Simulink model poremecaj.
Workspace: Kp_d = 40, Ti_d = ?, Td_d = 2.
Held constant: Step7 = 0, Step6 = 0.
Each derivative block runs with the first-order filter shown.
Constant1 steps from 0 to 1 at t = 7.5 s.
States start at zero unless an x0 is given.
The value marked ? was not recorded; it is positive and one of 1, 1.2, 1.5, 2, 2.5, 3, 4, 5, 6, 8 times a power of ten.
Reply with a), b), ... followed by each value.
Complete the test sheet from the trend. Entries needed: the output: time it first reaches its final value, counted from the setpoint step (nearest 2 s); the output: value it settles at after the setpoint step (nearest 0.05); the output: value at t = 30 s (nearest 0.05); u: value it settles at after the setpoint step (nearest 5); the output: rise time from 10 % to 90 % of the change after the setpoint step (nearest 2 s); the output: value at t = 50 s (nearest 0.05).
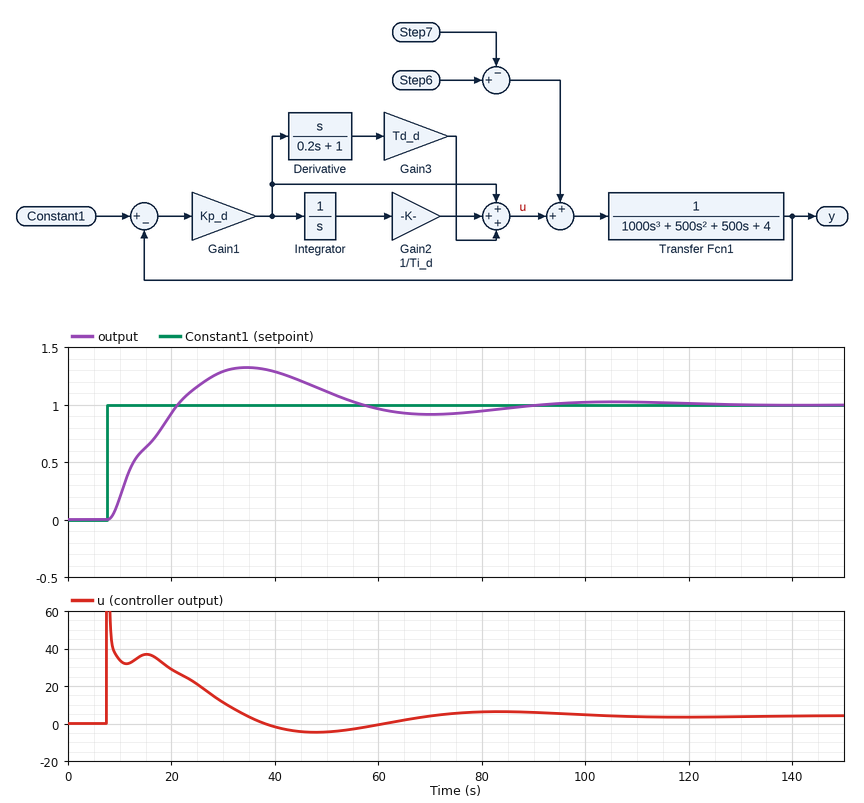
a) 14 s
b) 1.00
c) 1.30
d) 5
e) 10 s
f) 1.10
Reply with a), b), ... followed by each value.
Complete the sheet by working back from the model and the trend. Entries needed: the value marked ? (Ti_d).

a) 8
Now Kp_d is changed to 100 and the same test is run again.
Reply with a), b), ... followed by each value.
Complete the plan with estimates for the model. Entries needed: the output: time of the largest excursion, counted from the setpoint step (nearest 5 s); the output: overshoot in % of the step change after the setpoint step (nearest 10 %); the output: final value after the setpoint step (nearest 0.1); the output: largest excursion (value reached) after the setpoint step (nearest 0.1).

a) 15 s
b) 20 %
c) 1.0
d) 1.2
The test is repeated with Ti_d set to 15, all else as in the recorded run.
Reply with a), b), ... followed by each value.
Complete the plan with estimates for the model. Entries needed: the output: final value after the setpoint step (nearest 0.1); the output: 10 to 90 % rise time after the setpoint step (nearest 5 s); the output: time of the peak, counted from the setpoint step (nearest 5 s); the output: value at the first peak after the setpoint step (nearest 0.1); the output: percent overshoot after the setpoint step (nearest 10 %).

a) 1.0
b) 15 s
c) 35 s
d) 1.2
e) 20 %
